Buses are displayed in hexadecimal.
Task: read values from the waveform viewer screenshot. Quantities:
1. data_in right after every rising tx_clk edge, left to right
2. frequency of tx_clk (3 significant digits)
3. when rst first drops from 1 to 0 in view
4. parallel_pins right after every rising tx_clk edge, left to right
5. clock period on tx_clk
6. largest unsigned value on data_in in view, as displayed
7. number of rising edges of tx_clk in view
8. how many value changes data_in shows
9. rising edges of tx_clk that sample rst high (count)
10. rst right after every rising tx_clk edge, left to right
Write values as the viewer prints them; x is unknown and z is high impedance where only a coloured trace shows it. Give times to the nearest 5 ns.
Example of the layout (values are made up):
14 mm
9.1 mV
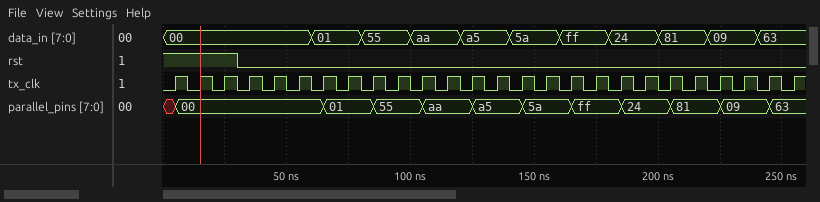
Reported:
00, 00, 00, 00, 00, 00, 01, 01, 55, 55, aa, aa, a5, a5, 5a, 5a, ff, ff, 24, 24, 81, 81, 09, 09, 63, 63
100 MHz
30 ns
00, 00, 00, 00, 00, 00, 01, 01, 55, 55, aa, aa, a5, a5, 5a, 5a, ff, ff, 24, 24, 81, 81, 09, 09, 63, 63
10 ns
ff
26
10
3
1 1 1 0 0 0 0 0 0 0 0 0 0 0 0 0 0 0 0 0 0 0 0 0 0 0
